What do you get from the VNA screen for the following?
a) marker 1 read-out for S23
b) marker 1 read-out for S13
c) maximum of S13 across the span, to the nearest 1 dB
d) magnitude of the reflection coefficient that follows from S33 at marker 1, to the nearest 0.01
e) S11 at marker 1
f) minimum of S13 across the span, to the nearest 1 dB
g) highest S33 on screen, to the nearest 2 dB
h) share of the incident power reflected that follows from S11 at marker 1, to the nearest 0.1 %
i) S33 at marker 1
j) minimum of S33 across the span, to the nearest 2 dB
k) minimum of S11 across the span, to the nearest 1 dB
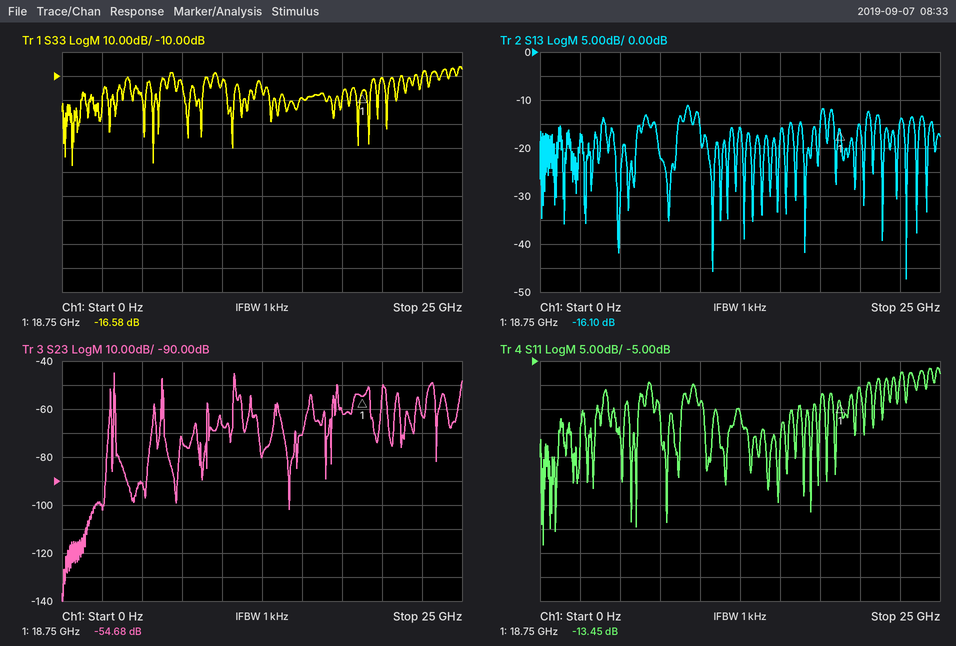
-54.68 dB
-16.10 dB
-11 dB
0.15
-13.45 dB
-47 dB
-6 dB
4.5 %
-16.58 dB
-48 dB
-43 dB
